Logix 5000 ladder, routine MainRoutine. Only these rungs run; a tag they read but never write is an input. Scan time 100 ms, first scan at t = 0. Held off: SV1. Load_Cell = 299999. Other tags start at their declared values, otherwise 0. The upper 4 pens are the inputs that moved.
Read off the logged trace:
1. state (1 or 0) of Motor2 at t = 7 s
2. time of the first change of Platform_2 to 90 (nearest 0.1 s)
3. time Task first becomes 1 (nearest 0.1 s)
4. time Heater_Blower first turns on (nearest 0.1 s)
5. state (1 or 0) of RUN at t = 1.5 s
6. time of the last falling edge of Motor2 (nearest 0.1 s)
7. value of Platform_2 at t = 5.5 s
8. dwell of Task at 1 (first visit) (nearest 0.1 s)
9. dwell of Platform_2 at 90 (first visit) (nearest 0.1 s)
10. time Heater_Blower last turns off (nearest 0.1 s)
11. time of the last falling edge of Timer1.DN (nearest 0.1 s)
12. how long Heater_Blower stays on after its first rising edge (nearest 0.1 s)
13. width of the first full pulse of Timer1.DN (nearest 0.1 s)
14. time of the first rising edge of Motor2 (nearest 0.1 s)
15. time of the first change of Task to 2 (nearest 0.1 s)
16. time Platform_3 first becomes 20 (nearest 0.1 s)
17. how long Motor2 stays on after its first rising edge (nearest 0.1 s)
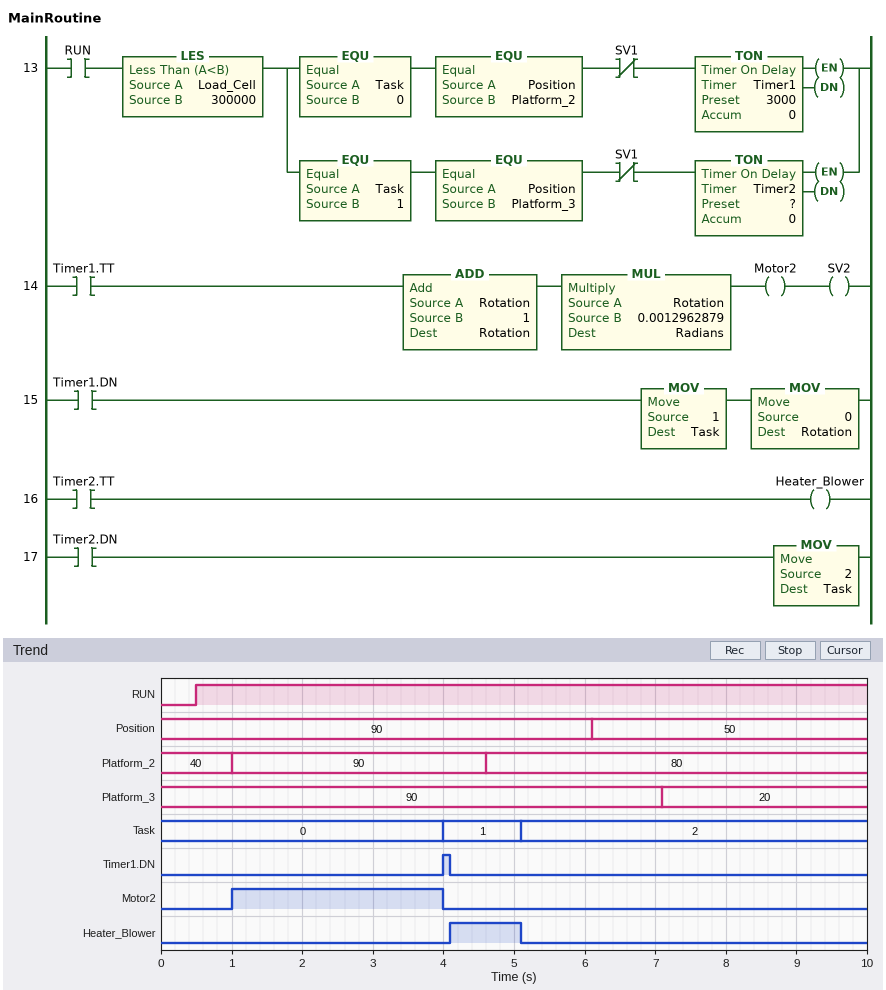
0
1.0 s
4.0 s
4.1 s
1
4.0 s
80
1.1 s
3.6 s
5.1 s
4.1 s
1.0 s
0.1 s
1.0 s
5.1 s
7.1 s
3.0 s
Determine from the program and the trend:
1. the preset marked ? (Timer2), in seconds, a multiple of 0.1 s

1.0 s
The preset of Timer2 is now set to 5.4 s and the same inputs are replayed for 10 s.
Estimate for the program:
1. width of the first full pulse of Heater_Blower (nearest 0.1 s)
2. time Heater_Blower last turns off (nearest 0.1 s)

2.0 s
6.1 s
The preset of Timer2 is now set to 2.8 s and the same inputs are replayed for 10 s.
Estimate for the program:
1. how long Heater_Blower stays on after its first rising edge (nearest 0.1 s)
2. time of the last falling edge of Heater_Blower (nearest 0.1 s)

2.0 s
6.1 s
